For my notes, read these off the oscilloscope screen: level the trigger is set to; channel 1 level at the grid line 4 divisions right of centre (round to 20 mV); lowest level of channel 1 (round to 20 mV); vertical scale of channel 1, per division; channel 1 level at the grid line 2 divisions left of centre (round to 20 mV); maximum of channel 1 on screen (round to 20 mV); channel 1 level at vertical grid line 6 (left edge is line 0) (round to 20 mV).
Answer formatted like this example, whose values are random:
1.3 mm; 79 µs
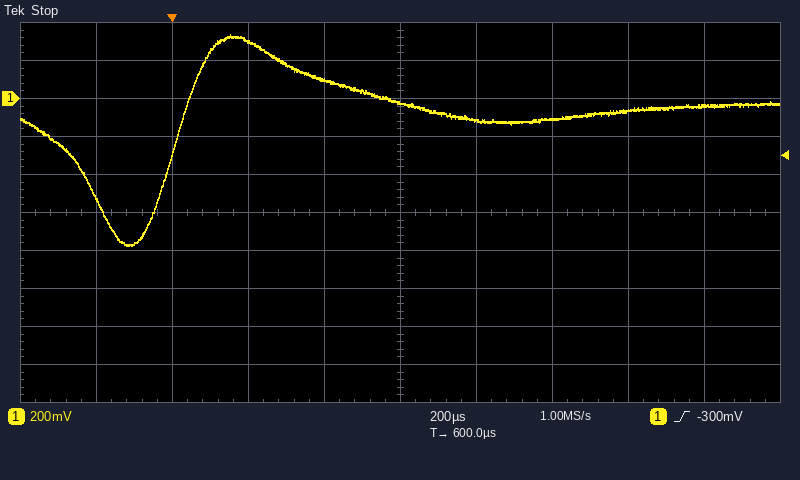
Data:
-300 mV; -40 mV; -780 mV; 200 mV; 300 mV; 340 mV; -120 mV
